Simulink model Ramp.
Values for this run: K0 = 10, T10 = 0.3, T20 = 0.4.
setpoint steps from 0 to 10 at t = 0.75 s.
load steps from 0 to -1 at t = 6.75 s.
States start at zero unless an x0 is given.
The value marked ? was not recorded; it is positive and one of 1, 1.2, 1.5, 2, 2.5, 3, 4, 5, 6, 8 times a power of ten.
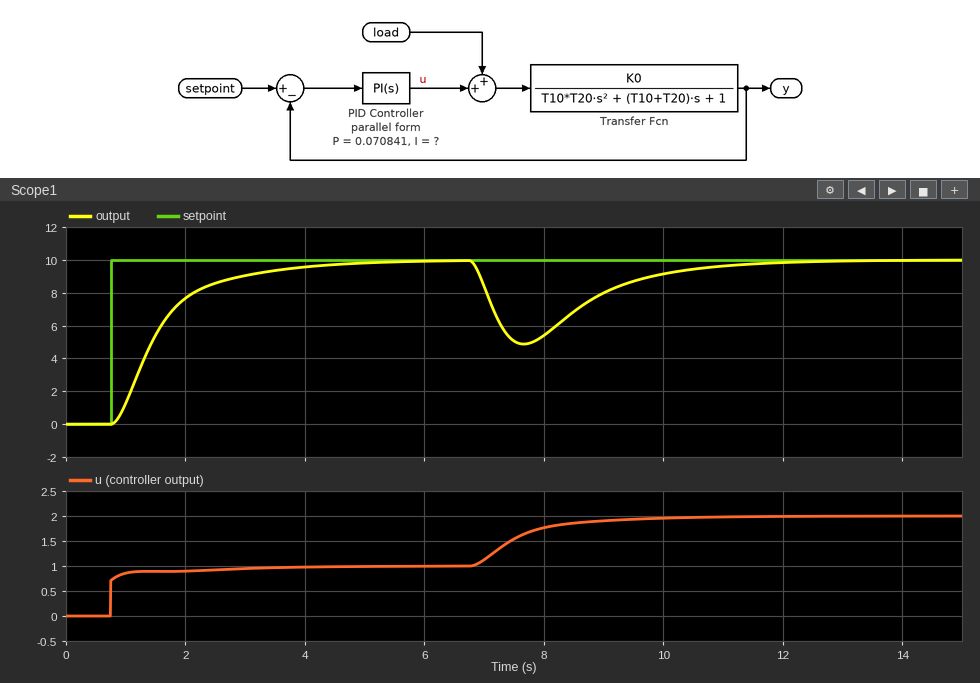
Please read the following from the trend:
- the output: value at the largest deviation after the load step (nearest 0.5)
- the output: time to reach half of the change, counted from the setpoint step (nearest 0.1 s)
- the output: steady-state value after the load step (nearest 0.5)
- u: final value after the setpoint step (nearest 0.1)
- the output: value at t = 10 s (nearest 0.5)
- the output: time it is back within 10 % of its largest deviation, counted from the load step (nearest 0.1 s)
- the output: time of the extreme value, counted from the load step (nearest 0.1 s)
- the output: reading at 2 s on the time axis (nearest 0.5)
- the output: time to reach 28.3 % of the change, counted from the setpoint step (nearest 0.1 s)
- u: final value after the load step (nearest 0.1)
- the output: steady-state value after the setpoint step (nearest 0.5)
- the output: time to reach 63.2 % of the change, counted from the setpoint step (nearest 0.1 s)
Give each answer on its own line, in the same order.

5.0
0.7 s
10.0
1.0
9.0
3.9 s
0.9 s
7.5
0.4 s
2.0
10.0
0.9 s
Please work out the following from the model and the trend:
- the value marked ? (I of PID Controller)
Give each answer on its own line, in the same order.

0.1
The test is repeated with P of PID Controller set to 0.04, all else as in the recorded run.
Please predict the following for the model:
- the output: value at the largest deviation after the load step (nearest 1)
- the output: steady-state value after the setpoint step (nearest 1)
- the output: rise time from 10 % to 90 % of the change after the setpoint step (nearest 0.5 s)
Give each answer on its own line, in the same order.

4
10
1.5 s
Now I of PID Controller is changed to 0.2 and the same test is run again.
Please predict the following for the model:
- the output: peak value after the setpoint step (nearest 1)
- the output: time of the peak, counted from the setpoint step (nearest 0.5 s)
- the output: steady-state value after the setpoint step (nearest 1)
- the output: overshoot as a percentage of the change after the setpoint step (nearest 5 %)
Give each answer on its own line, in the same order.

11
1.5 s
10
10 %
